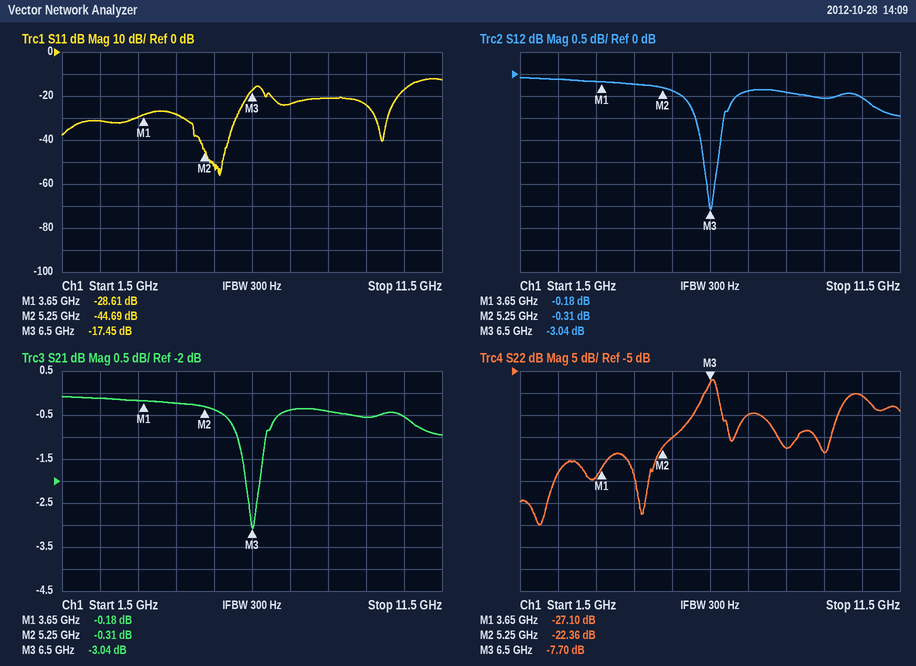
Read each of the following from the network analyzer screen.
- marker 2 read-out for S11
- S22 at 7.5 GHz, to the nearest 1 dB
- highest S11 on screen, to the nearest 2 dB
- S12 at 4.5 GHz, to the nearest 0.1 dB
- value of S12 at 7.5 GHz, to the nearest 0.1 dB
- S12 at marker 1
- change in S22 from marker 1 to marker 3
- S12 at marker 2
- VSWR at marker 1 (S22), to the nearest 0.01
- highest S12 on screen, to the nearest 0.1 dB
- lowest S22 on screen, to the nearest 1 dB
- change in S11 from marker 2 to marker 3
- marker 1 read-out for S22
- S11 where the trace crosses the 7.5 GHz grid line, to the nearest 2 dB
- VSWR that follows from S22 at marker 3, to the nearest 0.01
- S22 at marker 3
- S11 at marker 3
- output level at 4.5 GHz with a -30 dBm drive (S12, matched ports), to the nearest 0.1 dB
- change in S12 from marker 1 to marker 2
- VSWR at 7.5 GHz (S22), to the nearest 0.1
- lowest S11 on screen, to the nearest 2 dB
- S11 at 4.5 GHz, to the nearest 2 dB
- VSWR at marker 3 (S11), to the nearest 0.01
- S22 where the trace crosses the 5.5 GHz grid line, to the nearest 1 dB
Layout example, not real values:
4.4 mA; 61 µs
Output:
-44.69 dB; -15 dB; -12 dB; -0.2 dB; -0.4 dB; -0.18 dB; 19.40 dB; -0.31 dB; 1.09; -0.1 dB; -40 dB; 27.24 dB; -27.10 dB; -24 dB; 2.40; -7.70 dB; -17.45 dB; -30.2 dBm; -0.13 dB; 1.4; -56 dB; -28 dB; 1.31; -20 dB
